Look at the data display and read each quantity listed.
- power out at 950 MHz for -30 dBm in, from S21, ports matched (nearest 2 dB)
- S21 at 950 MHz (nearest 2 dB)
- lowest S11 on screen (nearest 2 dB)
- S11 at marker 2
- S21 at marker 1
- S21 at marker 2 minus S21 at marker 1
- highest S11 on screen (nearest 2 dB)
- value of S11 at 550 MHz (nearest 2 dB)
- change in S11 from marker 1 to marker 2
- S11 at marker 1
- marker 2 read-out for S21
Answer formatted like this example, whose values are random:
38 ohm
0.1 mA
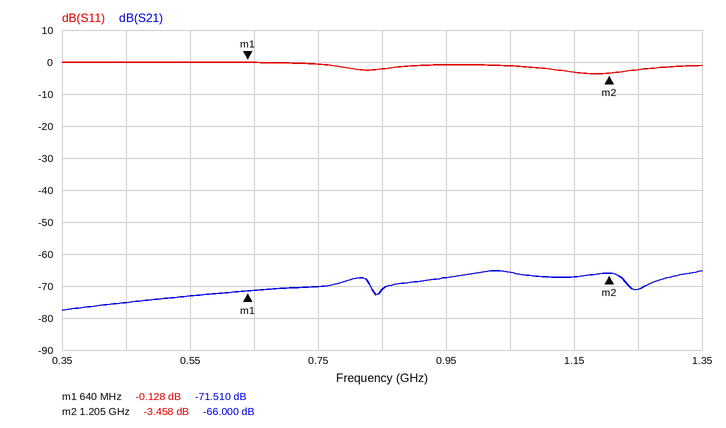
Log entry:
-98 dBm
-68 dB
-4 dB
-3.458 dB
-71.510 dB
5.510 dB
0 dB
0 dB
-3.330 dB
-0.128 dB
-66.000 dB
